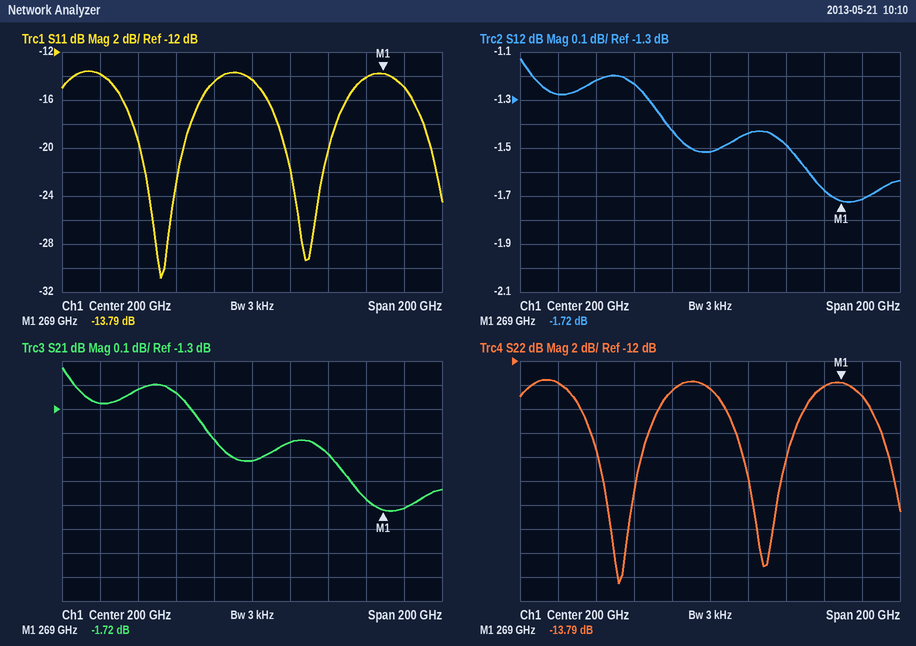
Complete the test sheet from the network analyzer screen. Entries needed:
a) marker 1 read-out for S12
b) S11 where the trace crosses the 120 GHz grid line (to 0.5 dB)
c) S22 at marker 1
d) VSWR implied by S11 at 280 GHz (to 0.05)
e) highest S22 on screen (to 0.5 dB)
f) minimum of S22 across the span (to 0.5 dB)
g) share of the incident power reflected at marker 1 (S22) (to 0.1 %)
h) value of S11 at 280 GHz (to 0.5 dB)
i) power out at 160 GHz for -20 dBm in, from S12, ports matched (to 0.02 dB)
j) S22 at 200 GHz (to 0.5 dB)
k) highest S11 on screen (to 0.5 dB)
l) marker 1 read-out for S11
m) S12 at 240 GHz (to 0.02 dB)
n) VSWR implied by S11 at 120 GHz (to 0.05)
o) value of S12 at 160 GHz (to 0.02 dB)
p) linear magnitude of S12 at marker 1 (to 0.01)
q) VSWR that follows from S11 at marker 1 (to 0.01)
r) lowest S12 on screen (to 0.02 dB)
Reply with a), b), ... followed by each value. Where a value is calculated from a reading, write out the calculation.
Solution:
a) -1.72 dB
b) -14.0 dB
c) -13.79 dB
d) |Γ| = 10^(-15/20) = 0.1778; VSWR = (1 + 0.1778)/(1 − 0.1778) ≈ 1.43, so 1.45 to the nearest 0.05
e) -13.5 dB
f) -30.5 dB
g) 10^(-13.79/10) ≈ 4.2 %
h) -15.0 dB
i) -20 dBm + (-1.24 dB) = -21.24 dBm
j) -14.5 dB
k) -13.5 dB
l) -13.79 dB
m) -1.48 dB
n) |Γ| = 10^(-14/20) = 0.1995; VSWR = (1 + 0.1995)/(1 − 0.1995) ≈ 1.50
o) -1.24 dB
p) 10^(-1.72/20) ≈ 0.82
q) (1 + 0.2044)/(1 − 0.2044) ≈ 1.51
r) -1.72 dB
